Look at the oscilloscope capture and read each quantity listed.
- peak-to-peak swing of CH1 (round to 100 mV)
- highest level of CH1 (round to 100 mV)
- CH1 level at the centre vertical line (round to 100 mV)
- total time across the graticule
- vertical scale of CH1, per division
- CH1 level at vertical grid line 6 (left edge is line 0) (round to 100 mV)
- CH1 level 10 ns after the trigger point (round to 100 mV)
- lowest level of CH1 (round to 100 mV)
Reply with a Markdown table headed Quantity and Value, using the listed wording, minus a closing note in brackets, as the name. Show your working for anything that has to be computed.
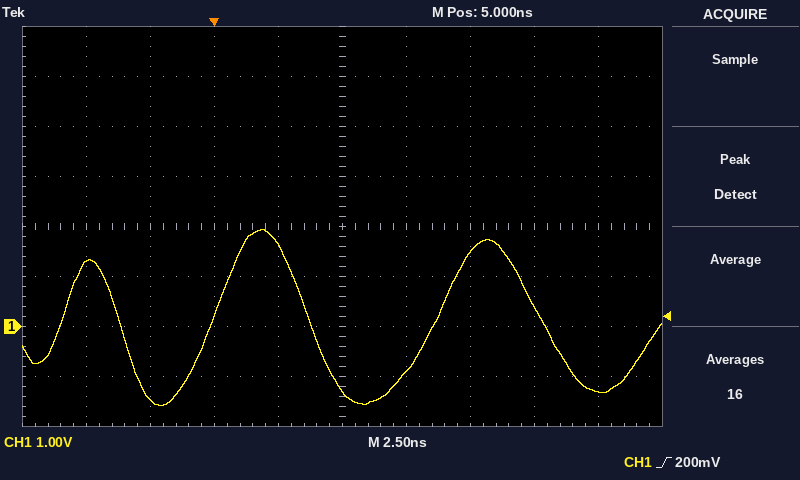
| Quantity | Value |
|---|---|
| peak-to-peak swing of CH1 | 1.9 V − (-1.6 V) = 3.5 V |
| highest level of CH1 | 1.9 V |
| CH1 level at the centre vertical line | -1.3 V |
| total time across the graticule | 25 ns |
| vertical scale of CH1, per division | 1 V |
| CH1 level at vertical grid line 6 (left edge is line 0) | -900 mV |
| CH1 level 10 ns after the trigger point | 1.5 V |
| lowest level of CH1 | -1.6 V |
